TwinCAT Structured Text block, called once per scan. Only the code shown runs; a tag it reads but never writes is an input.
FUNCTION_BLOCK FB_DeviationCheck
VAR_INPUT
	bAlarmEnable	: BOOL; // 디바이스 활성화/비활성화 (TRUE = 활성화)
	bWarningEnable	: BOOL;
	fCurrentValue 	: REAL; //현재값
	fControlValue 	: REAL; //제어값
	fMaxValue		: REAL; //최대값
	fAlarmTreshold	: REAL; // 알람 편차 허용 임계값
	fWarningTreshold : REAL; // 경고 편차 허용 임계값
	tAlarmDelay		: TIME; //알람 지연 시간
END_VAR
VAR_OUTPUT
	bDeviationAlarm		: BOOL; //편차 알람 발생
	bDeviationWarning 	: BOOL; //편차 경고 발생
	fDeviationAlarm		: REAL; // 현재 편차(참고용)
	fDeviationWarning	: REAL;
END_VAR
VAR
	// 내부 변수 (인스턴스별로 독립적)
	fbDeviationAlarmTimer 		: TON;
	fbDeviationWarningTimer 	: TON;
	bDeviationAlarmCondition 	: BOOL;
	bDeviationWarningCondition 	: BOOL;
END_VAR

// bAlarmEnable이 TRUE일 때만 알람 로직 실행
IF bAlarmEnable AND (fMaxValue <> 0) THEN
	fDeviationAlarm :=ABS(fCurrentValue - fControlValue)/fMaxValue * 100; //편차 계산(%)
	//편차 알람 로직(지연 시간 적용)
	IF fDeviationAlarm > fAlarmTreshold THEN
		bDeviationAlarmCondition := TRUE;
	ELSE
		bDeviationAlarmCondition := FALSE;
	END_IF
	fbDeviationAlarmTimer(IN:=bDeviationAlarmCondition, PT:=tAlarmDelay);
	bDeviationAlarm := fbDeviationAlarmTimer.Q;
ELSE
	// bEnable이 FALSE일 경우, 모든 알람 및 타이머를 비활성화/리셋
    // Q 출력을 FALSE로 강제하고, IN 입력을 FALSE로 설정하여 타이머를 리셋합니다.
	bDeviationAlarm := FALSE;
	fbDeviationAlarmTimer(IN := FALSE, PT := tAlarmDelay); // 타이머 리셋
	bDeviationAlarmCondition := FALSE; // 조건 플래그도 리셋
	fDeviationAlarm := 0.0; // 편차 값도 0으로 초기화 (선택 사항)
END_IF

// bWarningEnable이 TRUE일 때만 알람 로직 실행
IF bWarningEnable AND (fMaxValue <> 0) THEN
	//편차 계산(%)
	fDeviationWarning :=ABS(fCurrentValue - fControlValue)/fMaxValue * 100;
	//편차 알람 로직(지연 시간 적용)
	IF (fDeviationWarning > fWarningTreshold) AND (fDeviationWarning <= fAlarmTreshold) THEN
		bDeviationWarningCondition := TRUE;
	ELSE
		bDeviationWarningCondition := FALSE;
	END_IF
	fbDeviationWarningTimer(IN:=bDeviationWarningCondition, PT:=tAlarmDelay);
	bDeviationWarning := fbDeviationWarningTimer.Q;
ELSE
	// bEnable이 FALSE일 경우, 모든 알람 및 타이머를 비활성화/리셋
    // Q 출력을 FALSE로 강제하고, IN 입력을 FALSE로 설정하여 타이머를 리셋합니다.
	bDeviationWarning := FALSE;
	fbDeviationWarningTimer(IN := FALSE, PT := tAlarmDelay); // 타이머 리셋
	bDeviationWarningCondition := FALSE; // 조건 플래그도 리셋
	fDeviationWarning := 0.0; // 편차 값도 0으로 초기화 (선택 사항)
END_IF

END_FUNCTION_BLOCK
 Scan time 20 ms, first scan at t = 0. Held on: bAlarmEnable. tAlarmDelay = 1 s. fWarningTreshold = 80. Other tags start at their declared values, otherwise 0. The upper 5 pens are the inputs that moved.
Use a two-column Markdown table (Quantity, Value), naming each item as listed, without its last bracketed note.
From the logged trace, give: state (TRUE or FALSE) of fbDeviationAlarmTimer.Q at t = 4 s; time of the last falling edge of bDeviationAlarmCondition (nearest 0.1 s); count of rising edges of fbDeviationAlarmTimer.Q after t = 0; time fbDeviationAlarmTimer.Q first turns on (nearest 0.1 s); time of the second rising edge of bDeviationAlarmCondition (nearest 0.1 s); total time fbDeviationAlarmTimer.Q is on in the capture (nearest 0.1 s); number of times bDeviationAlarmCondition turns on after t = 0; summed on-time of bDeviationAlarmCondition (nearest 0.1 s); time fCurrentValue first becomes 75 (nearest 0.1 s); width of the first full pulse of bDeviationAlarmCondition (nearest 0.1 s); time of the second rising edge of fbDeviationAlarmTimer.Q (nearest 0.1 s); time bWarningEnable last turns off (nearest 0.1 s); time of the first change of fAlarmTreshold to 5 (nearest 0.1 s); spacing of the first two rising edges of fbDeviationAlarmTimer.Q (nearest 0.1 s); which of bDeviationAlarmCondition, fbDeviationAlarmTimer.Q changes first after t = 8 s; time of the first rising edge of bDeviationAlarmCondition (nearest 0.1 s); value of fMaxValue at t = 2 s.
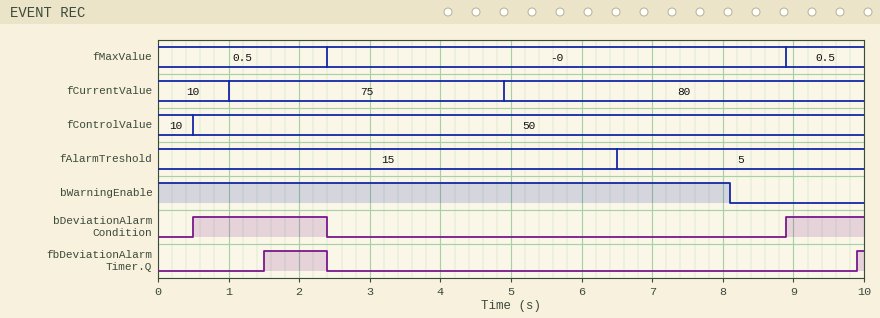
| Quantity | Value |
|---|---|
| state (TRUE or FALSE) of fbDeviationAlarmTimer.Q at t = 4 s | FALSE |
| time of the last falling edge of bDeviationAlarmCondition | 2.4 s |
| count of rising edges of fbDeviationAlarmTimer.Q after t = 0 | 2 |
| time fbDeviationAlarmTimer.Q first turns on | 1.5 s |
| time of the second rising edge of bDeviationAlarmCondition | 8.9 s |
| total time fbDeviationAlarmTimer.Q is on in the capture | 1.0 s |
| number of times bDeviationAlarmCondition turns on after t = 0 | 2 |
| summed on-time of bDeviationAlarmCondition | 3.0 s |
| time fCurrentValue first becomes 75 | 1.0 s |
| width of the first full pulse of bDeviationAlarmCondition | 1.9 s |
| time of the second rising edge of fbDeviationAlarmTimer.Q | 9.9 s |
| time bWarningEnable last turns off | 8.1 s |
| time of the first change of fAlarmTreshold to 5 | 6.5 s |
| spacing of the first two rising edges of fbDeviationAlarmTimer.Q | 8.4 s |
| which of bDeviationAlarmCondition, fbDeviationAlarmTimer.Q changes first after t = 8 s | bDeviationAlarmCondition |
| time of the first rising edge of bDeviationAlarmCondition | 0.5 s |
| value of fMaxValue at t = 2 s | 0.5 |
